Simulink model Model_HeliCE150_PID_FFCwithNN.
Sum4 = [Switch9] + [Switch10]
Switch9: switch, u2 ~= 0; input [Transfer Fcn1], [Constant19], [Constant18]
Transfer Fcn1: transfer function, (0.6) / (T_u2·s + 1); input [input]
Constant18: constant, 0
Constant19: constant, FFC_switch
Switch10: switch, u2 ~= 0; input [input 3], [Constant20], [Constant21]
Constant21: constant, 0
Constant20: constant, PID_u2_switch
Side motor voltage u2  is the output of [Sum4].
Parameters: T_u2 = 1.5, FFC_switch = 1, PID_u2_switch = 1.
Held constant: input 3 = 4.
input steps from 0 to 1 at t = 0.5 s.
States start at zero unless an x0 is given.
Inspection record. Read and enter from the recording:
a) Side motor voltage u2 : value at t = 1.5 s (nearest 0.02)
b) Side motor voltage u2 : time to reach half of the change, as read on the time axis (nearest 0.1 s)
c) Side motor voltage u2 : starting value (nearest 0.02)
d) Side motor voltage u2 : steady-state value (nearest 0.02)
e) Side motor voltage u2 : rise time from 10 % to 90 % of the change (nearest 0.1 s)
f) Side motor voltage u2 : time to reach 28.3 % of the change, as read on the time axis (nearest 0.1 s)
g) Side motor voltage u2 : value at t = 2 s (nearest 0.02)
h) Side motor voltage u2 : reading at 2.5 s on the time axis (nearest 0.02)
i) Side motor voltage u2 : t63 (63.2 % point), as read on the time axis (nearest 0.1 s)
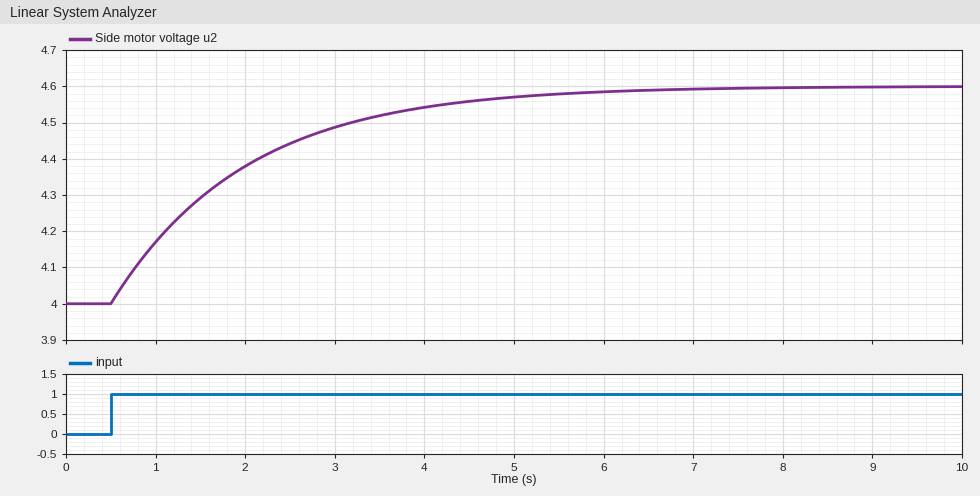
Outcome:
4.30
1.5 s
4.00
4.60
3.3 s
1.0 s
4.38
4.44
2.0 s
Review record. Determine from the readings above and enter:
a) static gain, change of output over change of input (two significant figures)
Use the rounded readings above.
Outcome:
0.60
